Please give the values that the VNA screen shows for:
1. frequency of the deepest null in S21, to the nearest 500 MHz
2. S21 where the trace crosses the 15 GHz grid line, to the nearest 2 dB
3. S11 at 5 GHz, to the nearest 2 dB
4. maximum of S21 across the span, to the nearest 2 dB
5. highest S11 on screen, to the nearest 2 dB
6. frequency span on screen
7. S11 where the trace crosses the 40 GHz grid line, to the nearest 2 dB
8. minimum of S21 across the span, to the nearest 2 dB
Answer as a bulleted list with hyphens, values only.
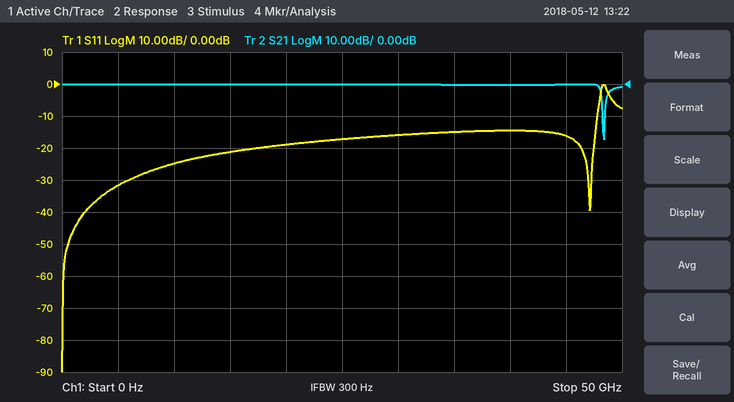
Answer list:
- 48.5 GHz
- 0 dB
- -32 dB
- 0 dB
- 0 dB
- 50 GHz
- -14 dB
- -18 dB
